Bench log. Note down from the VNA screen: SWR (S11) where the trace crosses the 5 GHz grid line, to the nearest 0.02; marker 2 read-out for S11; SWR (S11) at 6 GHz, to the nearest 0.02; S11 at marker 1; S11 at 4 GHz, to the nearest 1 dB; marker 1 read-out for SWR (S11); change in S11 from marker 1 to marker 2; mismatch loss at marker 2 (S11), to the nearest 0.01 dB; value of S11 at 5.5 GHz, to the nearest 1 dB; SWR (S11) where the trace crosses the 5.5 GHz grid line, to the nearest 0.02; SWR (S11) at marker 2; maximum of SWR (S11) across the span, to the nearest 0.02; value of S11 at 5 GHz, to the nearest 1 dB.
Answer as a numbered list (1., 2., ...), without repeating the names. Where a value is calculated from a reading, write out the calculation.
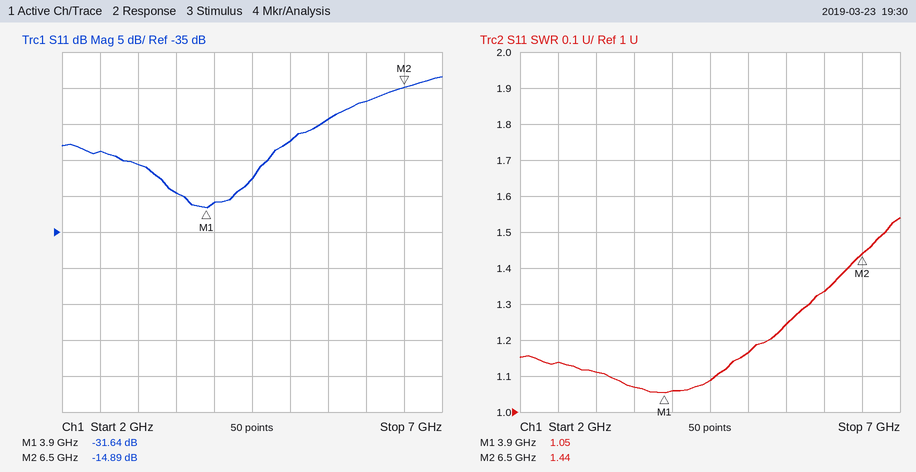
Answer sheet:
1. 1.16
2. -14.89 dB
3. 1.34
4. -31.64 dB
5. -31 dB
6. 1.05
7. -14.89 − (-31.64) = 16.75 dB
8. −10 log10(1 − 10^(-14.89/10)) ≈ 0.14 dB
9. -19 dB
10. 1.24
11. 1.44
12. 1.54
13. -22 dB
